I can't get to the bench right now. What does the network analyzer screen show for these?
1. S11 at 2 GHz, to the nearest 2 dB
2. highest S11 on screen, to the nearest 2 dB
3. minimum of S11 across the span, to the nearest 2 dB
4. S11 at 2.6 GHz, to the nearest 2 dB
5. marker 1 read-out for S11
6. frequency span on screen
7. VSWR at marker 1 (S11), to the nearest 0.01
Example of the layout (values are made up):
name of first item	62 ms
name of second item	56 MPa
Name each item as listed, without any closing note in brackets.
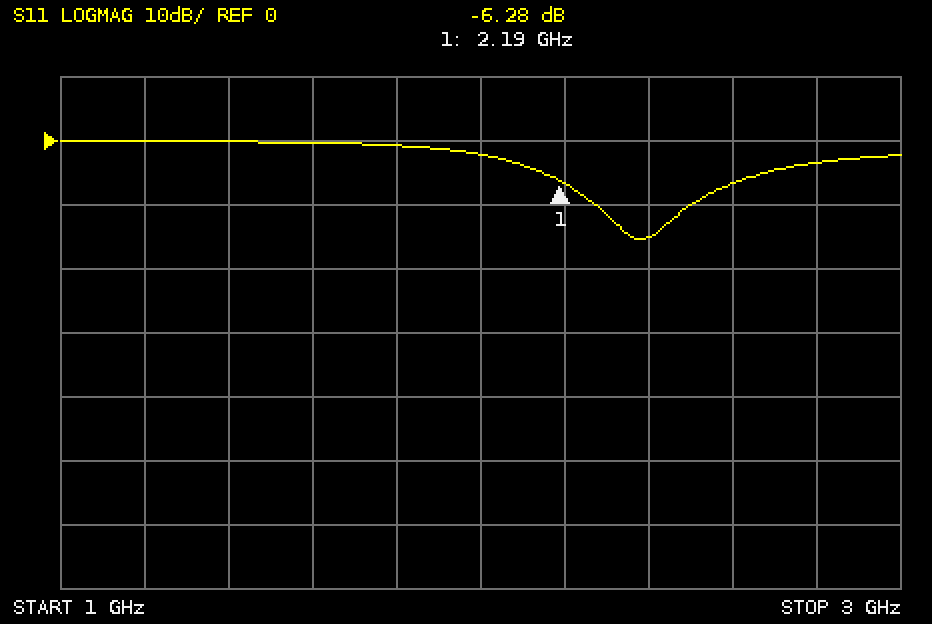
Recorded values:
S11 at 2 GHz, to the nearest 2 dB	-2 dB
highest S11 on screen, to the nearest 2 dB	0 dB
minimum of S11 across the span, to the nearest 2 dB	-16 dB
S11 at 2.6 GHz, to the nearest 2 dB	-6 dB
marker 1 read-out for S11	-6.28 dB
frequency span on screen	2 GHz
VSWR at marker 1 (S11), to the nearest 0.01	2.89
